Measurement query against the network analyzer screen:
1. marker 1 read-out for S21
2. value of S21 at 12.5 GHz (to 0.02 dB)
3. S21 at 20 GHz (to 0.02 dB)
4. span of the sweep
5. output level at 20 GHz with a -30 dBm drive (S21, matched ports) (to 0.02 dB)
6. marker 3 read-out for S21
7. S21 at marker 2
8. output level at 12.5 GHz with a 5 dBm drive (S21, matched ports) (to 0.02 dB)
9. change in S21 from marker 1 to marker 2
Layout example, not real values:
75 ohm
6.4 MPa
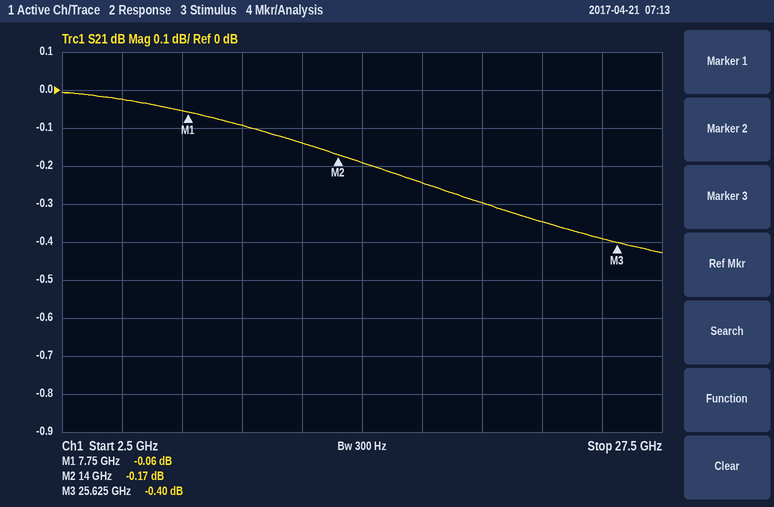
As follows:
-0.06 dB
-0.14 dB
-0.30 dB
25 GHz
-30.30 dBm
-0.40 dB
-0.17 dB
4.86 dBm
-0.11 dB
